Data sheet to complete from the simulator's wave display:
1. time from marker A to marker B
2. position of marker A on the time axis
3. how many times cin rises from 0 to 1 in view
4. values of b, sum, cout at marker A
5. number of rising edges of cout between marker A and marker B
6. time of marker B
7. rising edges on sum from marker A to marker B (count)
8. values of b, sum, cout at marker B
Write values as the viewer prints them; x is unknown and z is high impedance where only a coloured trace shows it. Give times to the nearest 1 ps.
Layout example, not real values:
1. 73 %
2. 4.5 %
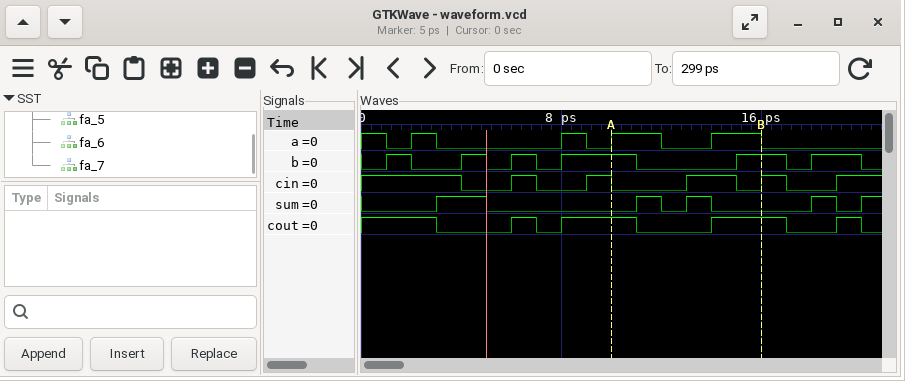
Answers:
1. 6 ps
2. 10 ps
3. 5
4. b=1, sum=0, cout=1
5. 1
6. 16 ps
7. 2
8. b=1, sum=0, cout=1
